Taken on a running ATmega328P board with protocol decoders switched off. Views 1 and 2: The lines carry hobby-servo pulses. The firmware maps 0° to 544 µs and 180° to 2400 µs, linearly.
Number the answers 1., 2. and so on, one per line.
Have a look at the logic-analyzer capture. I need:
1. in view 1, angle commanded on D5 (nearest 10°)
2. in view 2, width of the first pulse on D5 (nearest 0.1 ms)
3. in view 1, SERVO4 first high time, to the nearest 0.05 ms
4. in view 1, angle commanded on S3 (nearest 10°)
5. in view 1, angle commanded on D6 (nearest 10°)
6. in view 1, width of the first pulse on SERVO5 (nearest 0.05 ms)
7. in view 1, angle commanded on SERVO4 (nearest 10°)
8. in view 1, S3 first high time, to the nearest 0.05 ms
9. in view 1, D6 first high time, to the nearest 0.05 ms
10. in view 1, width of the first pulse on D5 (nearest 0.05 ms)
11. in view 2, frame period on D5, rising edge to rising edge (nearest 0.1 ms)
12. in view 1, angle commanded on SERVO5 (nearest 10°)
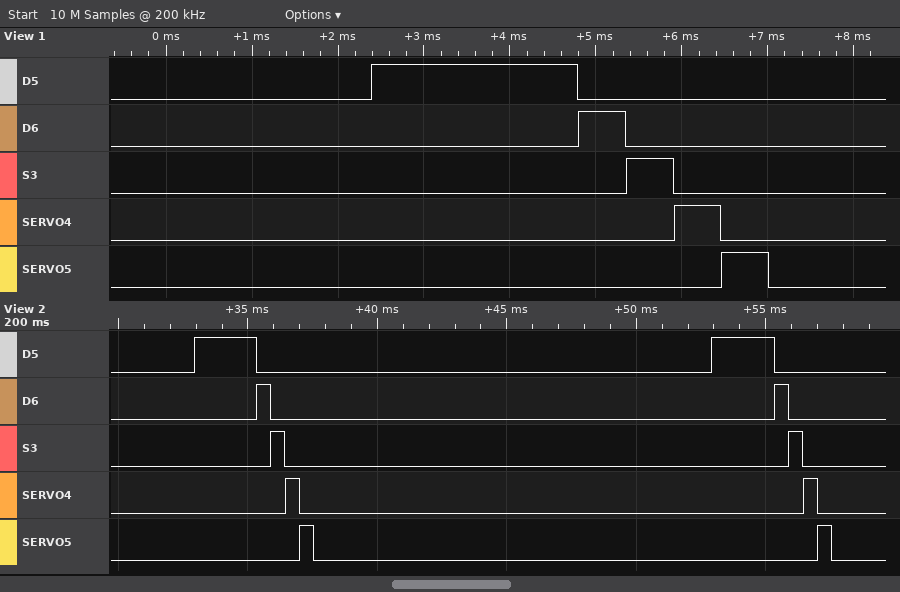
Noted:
1. 180°
2. 2.4 ms
3. 0.55 ms
4. 0°
5. 0°
6. 0.55 ms
7. 0°
8. 0.55 ms
9. 0.55 ms
10. 2.40 ms
11. 20.0 ms
12. 0°
